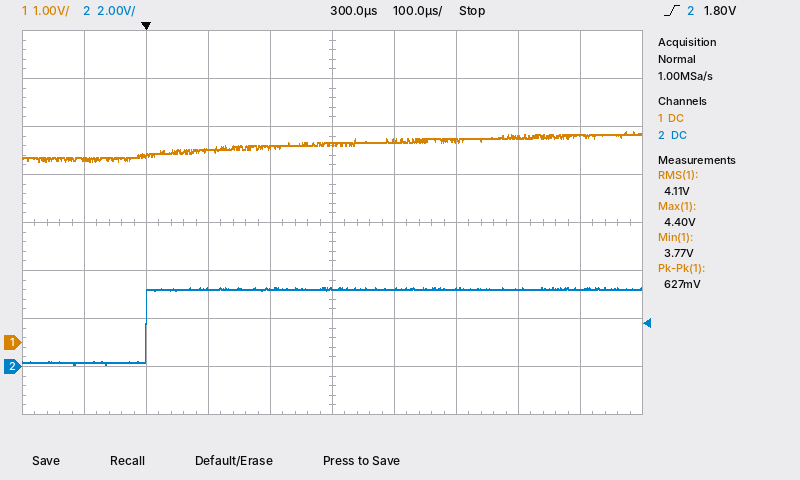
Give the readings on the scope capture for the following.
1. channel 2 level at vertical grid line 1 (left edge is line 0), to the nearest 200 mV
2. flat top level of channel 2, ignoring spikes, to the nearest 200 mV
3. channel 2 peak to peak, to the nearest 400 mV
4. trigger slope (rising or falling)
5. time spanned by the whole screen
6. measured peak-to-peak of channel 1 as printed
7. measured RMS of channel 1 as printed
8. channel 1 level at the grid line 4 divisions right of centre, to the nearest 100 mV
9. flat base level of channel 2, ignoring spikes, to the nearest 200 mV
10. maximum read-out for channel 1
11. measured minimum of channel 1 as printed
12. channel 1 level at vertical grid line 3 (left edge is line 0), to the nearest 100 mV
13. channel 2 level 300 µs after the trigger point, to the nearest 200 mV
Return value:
200 mV
3.2 V
3.2 V
rising
1 ms
627 mV
4.11 V
4.3 V
200 mV
4.40 V
3.77 V
4.0 V
3.2 V
